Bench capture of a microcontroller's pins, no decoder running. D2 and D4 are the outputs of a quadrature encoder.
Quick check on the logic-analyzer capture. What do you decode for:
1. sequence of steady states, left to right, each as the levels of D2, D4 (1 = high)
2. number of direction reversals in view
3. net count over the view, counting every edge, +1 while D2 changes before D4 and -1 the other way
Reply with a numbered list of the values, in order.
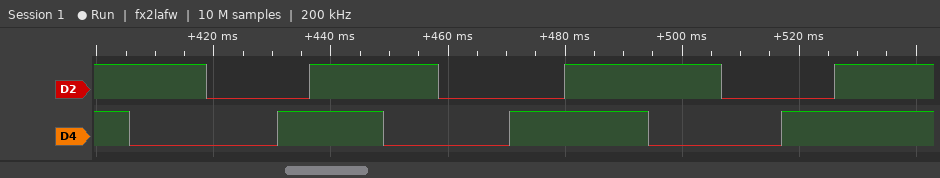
1. 11 10 00 01 11 10 00 01 11 10 00 01 11
2. 0
3. -12
